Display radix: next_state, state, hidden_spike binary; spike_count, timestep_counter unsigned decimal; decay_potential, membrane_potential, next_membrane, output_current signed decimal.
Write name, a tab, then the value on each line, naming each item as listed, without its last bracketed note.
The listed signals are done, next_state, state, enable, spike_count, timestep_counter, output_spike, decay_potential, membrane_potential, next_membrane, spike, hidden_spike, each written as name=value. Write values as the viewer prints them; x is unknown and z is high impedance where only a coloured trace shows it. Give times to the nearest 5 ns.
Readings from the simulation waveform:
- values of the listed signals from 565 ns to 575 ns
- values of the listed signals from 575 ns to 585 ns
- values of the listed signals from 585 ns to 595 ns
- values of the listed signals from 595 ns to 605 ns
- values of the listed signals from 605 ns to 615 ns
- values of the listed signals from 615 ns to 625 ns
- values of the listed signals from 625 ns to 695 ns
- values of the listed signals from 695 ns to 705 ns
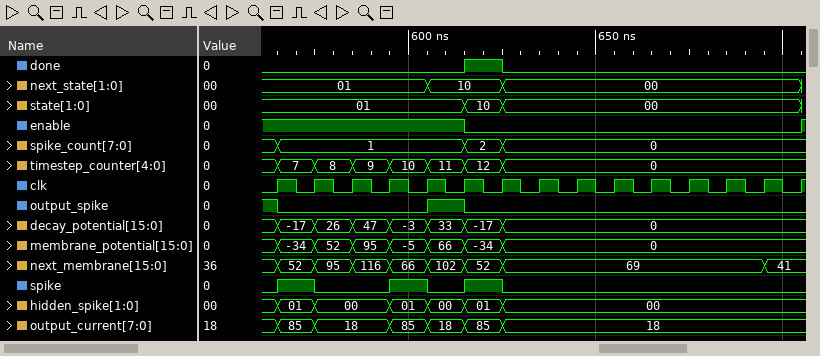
values of the listed signals from 565 ns to 575 ns	done=0, next_state=01, state=01, enable=1, spike_count=1, timestep_counter=7, output_spike=0, decay_potential=-17, membrane_potential=-34, next_membrane=52, spike=1, hidden_spike=01
values of the listed signals from 575 ns to 585 ns	done=0, next_state=01, state=01, enable=1, spike_count=1, timestep_counter=8, output_spike=0, decay_potential=26, membrane_potential=52, next_membrane=95, spike=0, hidden_spike=00
values of the listed signals from 585 ns to 595 ns	done=0, next_state=01, state=01, enable=1, spike_count=1, timestep_counter=9, output_spike=0, decay_potential=47, membrane_potential=95, next_membrane=116, spike=0, hidden_spike=00
values of the listed signals from 595 ns to 605 ns	done=0, next_state=01, state=01, enable=1, spike_count=1, timestep_counter=10, output_spike=0, decay_potential=-3, membrane_potential=-5, next_membrane=66, spike=1, hidden_spike=01
values of the listed signals from 605 ns to 615 ns	done=0, next_state=10, state=01, enable=1, spike_count=1, timestep_counter=11, output_spike=1, decay_potential=33, membrane_potential=66, next_membrane=102, spike=0, hidden_spike=00
values of the listed signals from 615 ns to 625 ns	done=1, next_state=10, state=10, enable=0, spike_count=2, timestep_counter=12, output_spike=0, decay_potential=-17, membrane_potential=-34, next_membrane=52, spike=1, hidden_spike=01
values of the listed signals from 625 ns to 695 ns	done=0, next_state=00, state=00, enable=0, spike_count=0, timestep_counter=0, output_spike=0, decay_potential=0, membrane_potential=0, next_membrane=69, spike=0, hidden_spike=00
values of the listed signals from 695 ns to 705 ns	done=0, next_state=00, state=00, enable=0, spike_count=0, timestep_counter=0, output_spike=0, decay_potential=0, membrane_potential=0, next_membrane=41, spike=0, hidden_spike=00
